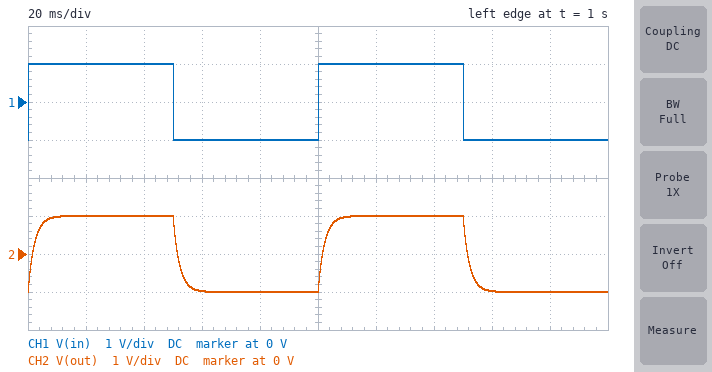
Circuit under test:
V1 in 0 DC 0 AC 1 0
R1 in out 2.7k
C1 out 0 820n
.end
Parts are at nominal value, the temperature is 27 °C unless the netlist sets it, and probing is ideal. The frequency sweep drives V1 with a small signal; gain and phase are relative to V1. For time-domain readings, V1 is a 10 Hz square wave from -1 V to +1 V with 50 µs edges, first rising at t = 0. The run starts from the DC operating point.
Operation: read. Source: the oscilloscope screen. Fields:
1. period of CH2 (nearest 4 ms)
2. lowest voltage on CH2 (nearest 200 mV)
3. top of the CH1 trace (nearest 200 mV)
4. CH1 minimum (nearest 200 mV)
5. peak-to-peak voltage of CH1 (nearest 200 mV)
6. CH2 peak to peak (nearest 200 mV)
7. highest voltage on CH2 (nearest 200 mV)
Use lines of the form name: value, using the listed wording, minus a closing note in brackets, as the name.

period of CH2: 100 ms
lowest voltage on CH2: -1.0 V
top of the CH1 trace: 1.0 V
CH1 minimum: -1.0 V
peak-to-peak voltage of CH1: 2.0 V
CH2 peak to peak: 2.0 V
highest voltage on CH2: 1.0 V
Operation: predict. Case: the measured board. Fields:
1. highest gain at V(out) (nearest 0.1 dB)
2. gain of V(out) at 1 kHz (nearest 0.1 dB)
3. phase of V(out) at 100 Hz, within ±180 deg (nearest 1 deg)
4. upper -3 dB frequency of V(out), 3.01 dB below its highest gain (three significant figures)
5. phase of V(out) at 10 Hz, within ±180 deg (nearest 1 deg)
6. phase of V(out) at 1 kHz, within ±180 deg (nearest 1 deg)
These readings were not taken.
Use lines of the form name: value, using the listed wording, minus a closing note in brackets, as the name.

highest gain at V(out): 0 dB
gain of V(out) at 1 kHz: -22.9 dB
phase of V(out) at 100 Hz, within ±180 deg: -54 deg
upper -3 dB frequency of V(out), 3.01 dB below its highest gain: 71.9 Hz
phase of V(out) at 10 Hz, within ±180 deg: -8 deg
phase of V(out) at 1 kHz, within ±180 deg: -86 deg
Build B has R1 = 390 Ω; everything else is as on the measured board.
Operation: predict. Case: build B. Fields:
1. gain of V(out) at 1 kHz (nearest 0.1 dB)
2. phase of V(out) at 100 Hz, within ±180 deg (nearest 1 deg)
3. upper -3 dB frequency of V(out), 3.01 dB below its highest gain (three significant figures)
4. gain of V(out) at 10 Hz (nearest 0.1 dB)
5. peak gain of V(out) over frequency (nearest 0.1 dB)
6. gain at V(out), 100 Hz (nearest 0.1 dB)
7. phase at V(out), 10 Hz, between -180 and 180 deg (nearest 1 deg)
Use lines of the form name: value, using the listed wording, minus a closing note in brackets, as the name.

gain of V(out) at 1 kHz: -7.0 dB
phase of V(out) at 100 Hz, within ±180 deg: -11 deg
upper -3 dB frequency of V(out), 3.01 dB below its highest gain: 498 Hz
gain of V(out) at 10 Hz: 0 dB
peak gain of V(out) over frequency: 0 dB
gain at V(out), 100 Hz: -0.2 dB
phase at V(out), 10 Hz, between -180 and 180 deg: -1 deg
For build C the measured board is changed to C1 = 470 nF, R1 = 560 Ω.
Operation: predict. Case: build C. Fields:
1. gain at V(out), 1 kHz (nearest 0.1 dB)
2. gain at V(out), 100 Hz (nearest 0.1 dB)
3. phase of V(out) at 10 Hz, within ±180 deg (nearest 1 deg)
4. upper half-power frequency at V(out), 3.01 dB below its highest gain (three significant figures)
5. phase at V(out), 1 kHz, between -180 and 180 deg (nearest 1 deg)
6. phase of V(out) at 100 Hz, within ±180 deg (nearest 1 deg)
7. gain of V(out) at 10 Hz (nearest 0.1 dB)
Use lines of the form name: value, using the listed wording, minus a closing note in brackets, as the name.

gain at V(out), 1 kHz: -5.7 dB
gain at V(out), 100 Hz: -0.1 dB
phase of V(out) at 10 Hz, within ±180 deg: -1 deg
upper half-power frequency at V(out), 3.01 dB below its highest gain: 605 Hz
phase at V(out), 1 kHz, between -180 and 180 deg: -59 deg
phase of V(out) at 100 Hz, within ±180 deg: -9 deg
gain of V(out) at 10 Hz: 0 dB
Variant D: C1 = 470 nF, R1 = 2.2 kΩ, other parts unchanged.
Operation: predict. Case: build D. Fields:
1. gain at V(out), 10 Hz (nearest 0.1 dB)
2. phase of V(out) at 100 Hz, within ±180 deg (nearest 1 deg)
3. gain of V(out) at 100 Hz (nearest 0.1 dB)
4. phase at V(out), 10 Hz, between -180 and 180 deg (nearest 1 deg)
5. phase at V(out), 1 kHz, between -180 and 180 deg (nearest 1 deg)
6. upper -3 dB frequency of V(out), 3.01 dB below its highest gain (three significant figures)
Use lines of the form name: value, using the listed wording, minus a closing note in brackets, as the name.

gain at V(out), 10 Hz: 0 dB
phase of V(out) at 100 Hz, within ±180 deg: -33 deg
gain of V(out) at 100 Hz: -1.5 dB
phase at V(out), 10 Hz, between -180 and 180 deg: -4 deg
phase at V(out), 1 kHz, between -180 and 180 deg: -81 deg
upper -3 dB frequency of V(out), 3.01 dB below its highest gain: 154 Hz
